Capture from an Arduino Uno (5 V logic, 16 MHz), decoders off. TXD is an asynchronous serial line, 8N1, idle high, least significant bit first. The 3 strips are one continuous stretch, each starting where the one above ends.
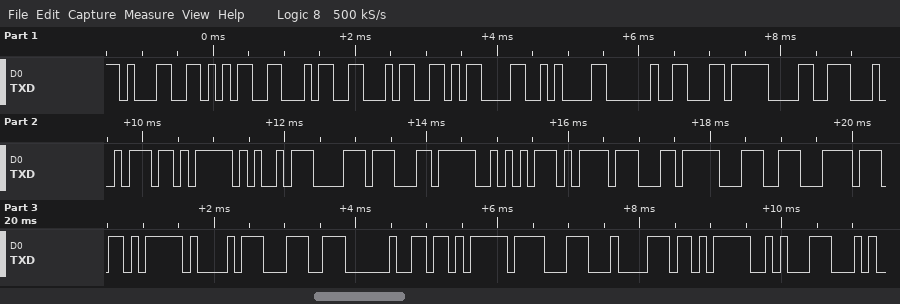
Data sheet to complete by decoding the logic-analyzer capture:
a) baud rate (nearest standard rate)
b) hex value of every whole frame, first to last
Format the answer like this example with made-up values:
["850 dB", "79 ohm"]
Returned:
["9600 baud", "31 35 34 34 0D 0A 20 EC 98 A4 EB A5 B8 EC AA BD EC 9C BC EB A1 9C 20 EB 8F 84 EB 8A"]
